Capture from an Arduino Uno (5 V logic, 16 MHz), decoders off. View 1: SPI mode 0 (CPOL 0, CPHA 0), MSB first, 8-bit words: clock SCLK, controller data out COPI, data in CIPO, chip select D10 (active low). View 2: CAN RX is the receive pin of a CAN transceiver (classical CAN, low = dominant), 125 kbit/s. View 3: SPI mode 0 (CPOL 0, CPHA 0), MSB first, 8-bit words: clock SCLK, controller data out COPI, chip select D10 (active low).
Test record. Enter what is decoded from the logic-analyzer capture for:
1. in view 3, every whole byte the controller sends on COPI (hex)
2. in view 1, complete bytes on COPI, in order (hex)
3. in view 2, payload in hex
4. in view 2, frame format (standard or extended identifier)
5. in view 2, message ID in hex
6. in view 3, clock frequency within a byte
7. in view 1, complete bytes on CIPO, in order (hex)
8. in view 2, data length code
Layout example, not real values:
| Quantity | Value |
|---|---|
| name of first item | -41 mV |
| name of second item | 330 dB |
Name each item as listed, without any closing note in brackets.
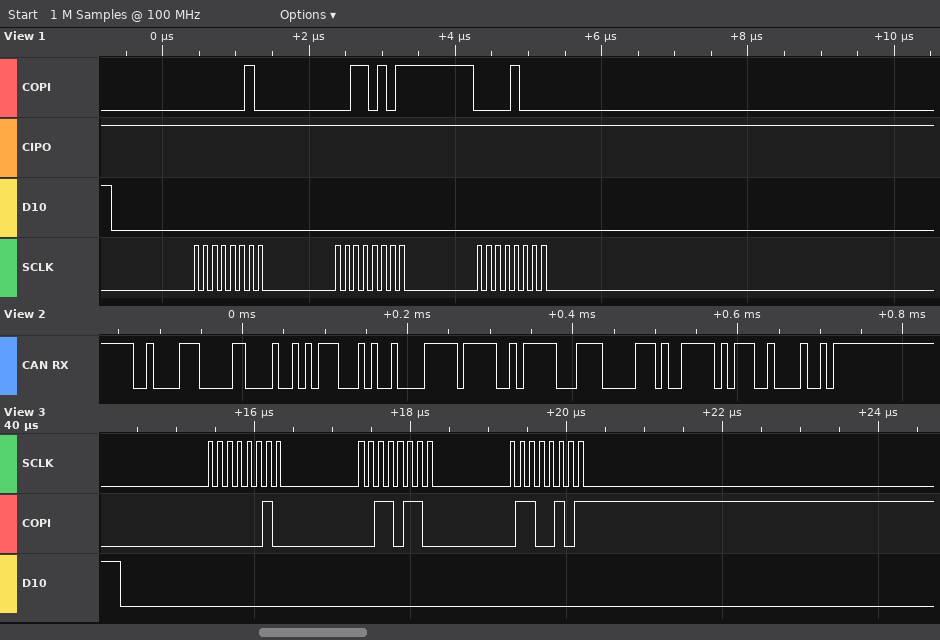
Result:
| Quantity | Value |
|---|---|
| in view 3, every whole byte the controller sends on COPI | 02 36 65 |
| in view 1, complete bytes on COPI, in order | 02 35 08 |
| in view 2, payload in hex | 4A E2 90 FF D7 CF 06 9F |
| in view 2, frame format | standard |
| in view 2, message ID in hex | 0x21C |
| in view 3, clock frequency within a byte | 8 MHz |
| in view 1, complete bytes on CIPO, in order | FF FF FF |
| in view 2, data length code | 8 |
